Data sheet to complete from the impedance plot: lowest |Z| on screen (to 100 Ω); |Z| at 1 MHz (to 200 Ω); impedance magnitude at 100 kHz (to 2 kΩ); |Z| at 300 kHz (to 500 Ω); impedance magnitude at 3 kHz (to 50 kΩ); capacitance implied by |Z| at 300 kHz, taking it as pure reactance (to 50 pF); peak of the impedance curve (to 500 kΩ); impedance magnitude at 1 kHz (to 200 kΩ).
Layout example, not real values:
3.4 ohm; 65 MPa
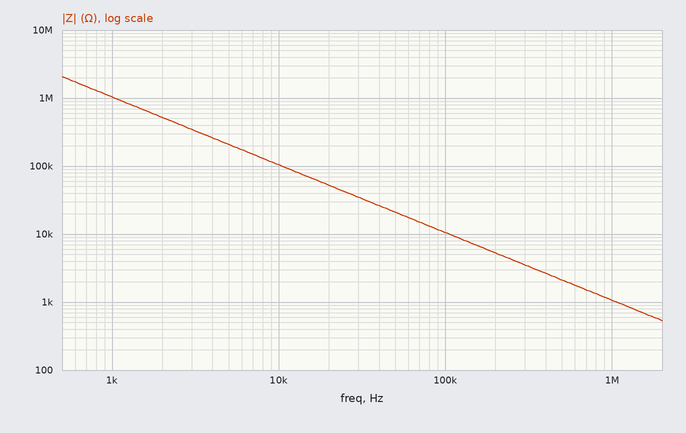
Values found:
500 Ω; 1.0 kΩ; 10 kΩ; 3.5 kΩ; 350 kΩ; 150 pF; 2.0 MΩ; 1.0 MΩ
